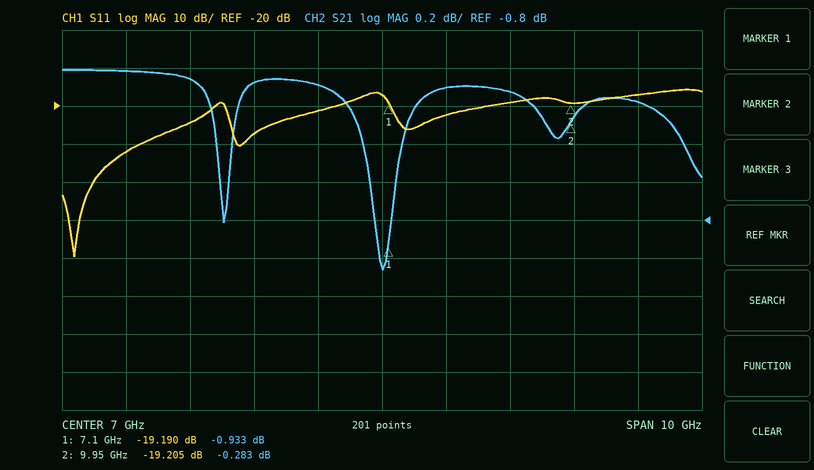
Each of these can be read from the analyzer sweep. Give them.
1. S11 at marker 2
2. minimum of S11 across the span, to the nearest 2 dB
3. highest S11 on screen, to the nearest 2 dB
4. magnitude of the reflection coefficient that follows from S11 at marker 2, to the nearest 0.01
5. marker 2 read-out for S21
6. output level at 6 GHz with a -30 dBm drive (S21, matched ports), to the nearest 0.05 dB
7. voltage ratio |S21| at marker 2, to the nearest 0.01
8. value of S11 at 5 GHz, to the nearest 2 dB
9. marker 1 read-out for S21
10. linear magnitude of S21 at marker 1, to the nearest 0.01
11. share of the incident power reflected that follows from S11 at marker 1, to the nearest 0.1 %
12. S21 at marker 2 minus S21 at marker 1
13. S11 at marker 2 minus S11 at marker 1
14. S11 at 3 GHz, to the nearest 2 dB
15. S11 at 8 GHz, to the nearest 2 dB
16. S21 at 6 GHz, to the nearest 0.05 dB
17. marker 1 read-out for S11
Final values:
-19.205 dB
-60 dB
-16 dB
0.11
-0.283 dB
-30.10 dBm
0.97
-28 dB
-0.933 dB
0.90
1.2 %
0.650 dB
-0.015 dB
-32 dB
-22 dB
-0.10 dB
-19.190 dB
